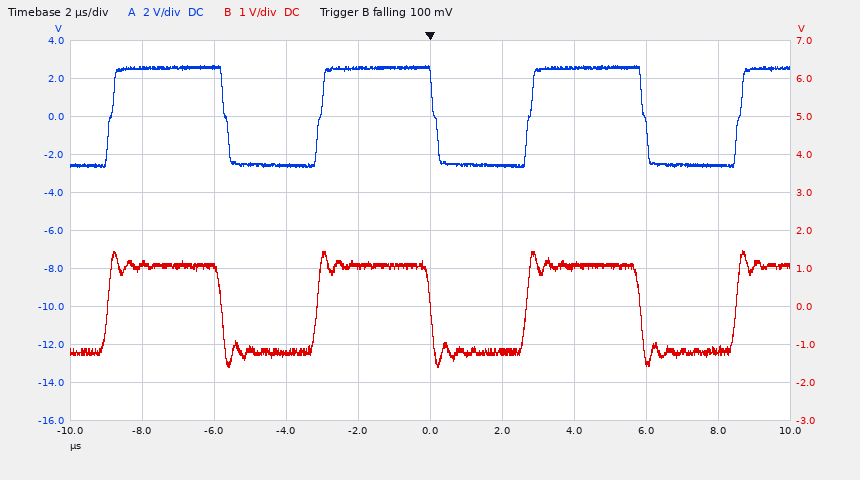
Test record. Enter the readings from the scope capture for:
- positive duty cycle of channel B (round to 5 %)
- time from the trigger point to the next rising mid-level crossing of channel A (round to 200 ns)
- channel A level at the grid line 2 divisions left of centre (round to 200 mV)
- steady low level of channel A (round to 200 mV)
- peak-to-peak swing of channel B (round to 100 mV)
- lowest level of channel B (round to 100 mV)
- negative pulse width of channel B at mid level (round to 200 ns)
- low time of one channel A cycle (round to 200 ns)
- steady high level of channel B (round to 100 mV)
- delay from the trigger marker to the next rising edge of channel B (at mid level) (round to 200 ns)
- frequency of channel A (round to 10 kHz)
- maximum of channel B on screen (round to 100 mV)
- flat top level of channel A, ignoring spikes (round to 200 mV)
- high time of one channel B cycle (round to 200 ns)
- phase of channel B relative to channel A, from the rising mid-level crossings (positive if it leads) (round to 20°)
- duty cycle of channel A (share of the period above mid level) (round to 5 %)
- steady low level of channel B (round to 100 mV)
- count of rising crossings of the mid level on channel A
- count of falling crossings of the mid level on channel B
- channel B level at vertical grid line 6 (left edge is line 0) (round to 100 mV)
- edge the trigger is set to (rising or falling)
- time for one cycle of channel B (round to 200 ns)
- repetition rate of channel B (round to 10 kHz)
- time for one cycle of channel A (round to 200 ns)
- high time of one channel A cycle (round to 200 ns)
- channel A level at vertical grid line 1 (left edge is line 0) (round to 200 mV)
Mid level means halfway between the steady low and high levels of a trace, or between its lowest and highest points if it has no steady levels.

55 %
2.8 µs
-2.6 V
-2.6 V
3.1 V
-1.6 V
2.6 µs
2.6 µs
1.1 V
2.6 µs
170 kHz
1.5 V
2.6 V
3.2 µs
0°
55 %
-1.2 V
4
3
-1.2 V
falling
5.8 µs
170 kHz
5.8 µs
3.2 µs
2.6 V
